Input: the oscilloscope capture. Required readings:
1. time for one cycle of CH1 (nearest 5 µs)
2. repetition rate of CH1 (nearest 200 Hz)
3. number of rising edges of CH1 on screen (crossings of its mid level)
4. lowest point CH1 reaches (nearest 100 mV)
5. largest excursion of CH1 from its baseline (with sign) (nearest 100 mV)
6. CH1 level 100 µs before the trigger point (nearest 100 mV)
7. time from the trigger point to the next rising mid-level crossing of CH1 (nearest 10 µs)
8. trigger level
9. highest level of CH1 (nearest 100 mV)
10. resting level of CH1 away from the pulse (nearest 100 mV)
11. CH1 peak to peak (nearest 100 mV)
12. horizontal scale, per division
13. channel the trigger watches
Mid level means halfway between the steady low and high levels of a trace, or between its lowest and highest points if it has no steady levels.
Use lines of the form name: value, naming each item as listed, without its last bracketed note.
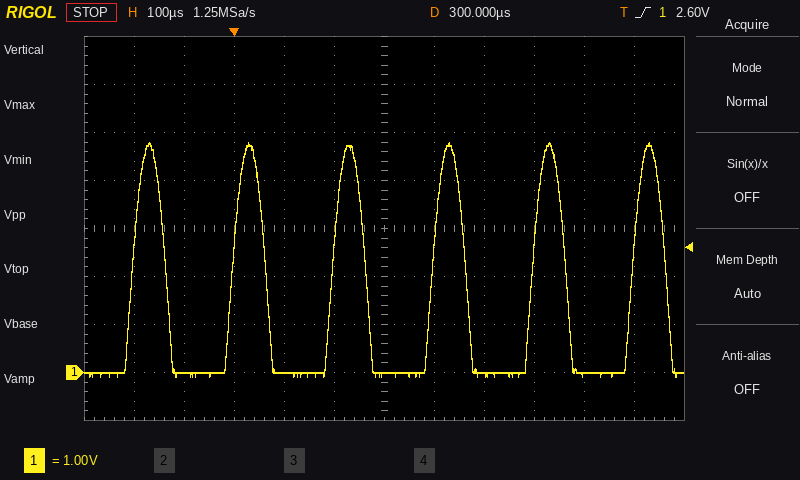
time for one cycle of CH1: 200 µs
repetition rate of CH1: 5.0 kHz
number of rising edges of CH1 on screen: 6
lowest point CH1 reaches: -100 mV
largest excursion of CH1 from its baseline (with sign): +4.8 V
CH1 level 100 µs before the trigger point: 0.0 V
time from the trigger point to the next rising mid-level crossing of CH1: 200 µs
trigger level: 2.60 V
highest level of CH1: 4.8 V
resting level of CH1 away from the pulse: 0.0 V
CH1 peak to peak: 4.9 V
horizontal scale, per division: 100 µs
channel the trigger watches: CH1
